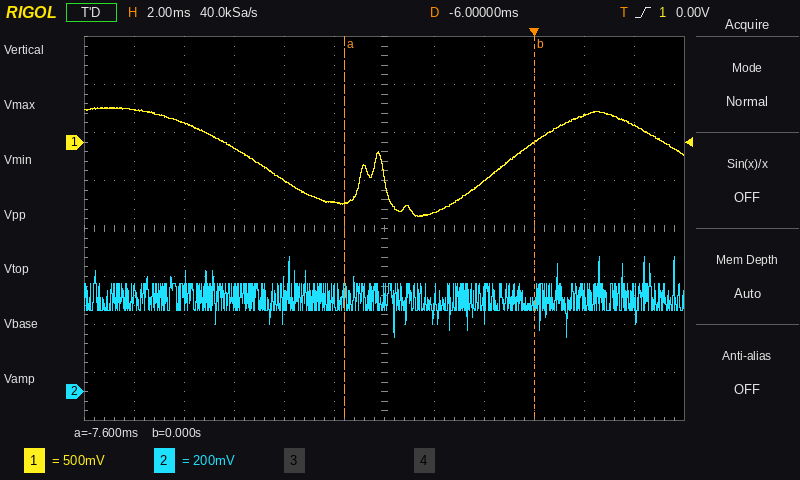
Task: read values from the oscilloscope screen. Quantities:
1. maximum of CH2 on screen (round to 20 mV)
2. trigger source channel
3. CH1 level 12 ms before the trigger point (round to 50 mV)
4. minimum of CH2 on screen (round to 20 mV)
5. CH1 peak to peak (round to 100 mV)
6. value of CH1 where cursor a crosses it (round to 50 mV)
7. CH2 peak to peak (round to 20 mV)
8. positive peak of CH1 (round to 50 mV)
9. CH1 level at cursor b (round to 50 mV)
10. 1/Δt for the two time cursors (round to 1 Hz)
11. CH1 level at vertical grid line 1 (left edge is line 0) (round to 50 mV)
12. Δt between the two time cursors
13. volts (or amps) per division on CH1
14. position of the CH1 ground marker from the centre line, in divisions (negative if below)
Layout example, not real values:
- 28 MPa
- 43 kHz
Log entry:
- 560 mV
- CH1
- -50 mV
- 220 mV
- 1.10 V
- -650 mV
- 340 mV
- 350 mV
- 0 mV
- 132 Hz
- 350 mV
- 7.6 ms
- 500 mV
- +1.8 div
